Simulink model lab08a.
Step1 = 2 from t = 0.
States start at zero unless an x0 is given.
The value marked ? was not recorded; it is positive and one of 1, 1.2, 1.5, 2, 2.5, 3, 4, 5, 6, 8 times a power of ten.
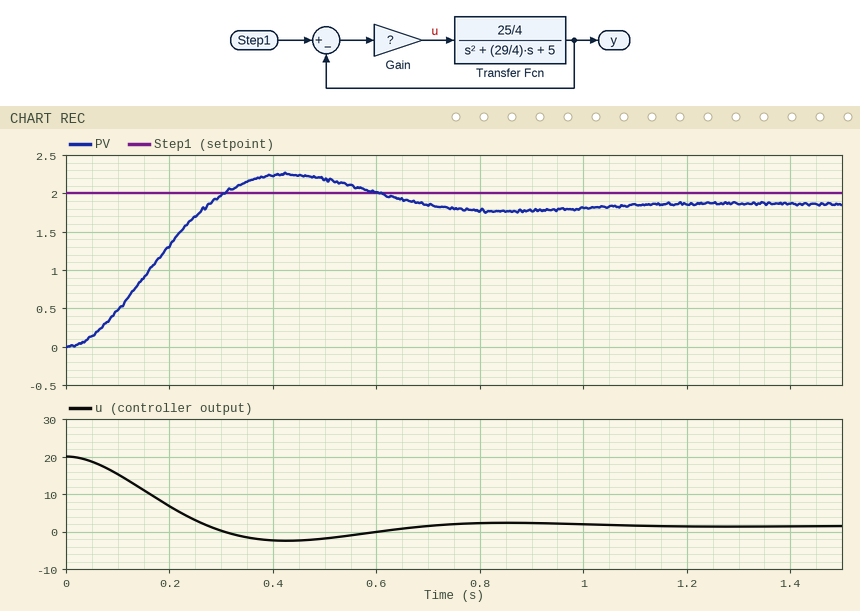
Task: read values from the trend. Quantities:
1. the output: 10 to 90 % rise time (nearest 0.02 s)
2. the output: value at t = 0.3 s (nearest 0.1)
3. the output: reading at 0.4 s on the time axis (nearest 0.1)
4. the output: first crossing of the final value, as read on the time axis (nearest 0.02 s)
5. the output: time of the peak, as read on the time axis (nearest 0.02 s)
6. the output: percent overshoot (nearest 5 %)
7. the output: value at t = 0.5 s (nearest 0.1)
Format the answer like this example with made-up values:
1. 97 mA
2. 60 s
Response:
1. 0.18 s
2. 2.0
3. 2.2
4. 0.28 s
5. 0.42 s
6. 20 %
7. 2.2
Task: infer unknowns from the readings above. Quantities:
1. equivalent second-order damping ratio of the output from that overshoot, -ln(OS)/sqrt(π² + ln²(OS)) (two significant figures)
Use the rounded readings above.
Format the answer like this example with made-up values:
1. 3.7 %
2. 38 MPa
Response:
1. 0.46
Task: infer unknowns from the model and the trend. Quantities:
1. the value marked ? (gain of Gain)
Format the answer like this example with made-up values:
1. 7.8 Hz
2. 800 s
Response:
1. 10
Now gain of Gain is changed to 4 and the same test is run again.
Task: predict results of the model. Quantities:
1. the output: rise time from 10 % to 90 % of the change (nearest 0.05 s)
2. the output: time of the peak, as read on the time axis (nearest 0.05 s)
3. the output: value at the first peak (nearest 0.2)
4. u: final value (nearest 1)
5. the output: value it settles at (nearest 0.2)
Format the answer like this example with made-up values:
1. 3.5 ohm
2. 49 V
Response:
1. 0.35 s
2. 0.75 s
3. 1.8
4. 1
5. 1.6
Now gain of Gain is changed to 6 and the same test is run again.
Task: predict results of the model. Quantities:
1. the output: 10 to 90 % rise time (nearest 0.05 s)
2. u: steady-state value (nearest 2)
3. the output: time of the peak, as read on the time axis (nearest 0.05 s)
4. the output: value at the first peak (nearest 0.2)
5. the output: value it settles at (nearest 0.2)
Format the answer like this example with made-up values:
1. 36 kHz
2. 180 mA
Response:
1. 0.25 s
2. 2
3. 0.60 s
4. 2.0
5. 1.8
